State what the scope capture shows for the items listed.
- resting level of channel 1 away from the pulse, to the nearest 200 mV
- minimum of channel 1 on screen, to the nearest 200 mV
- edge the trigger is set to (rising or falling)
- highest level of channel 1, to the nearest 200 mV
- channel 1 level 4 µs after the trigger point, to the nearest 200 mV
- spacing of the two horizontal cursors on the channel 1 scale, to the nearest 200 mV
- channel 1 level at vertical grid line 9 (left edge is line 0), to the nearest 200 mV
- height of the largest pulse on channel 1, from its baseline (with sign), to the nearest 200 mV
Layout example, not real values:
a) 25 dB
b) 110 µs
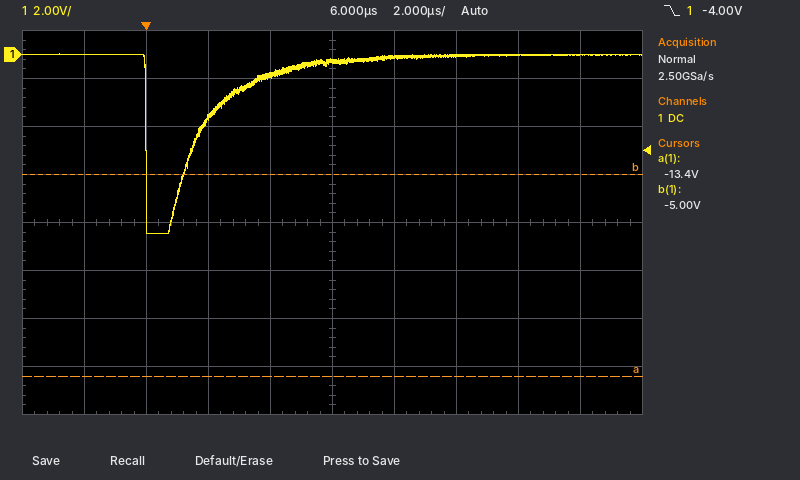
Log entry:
a) 0.0 V
b) -7.4 V
c) falling
d) 0.0 V
e) -800 mV
f) 8.4 V
g) 0.0 V
h) -7.4 V
